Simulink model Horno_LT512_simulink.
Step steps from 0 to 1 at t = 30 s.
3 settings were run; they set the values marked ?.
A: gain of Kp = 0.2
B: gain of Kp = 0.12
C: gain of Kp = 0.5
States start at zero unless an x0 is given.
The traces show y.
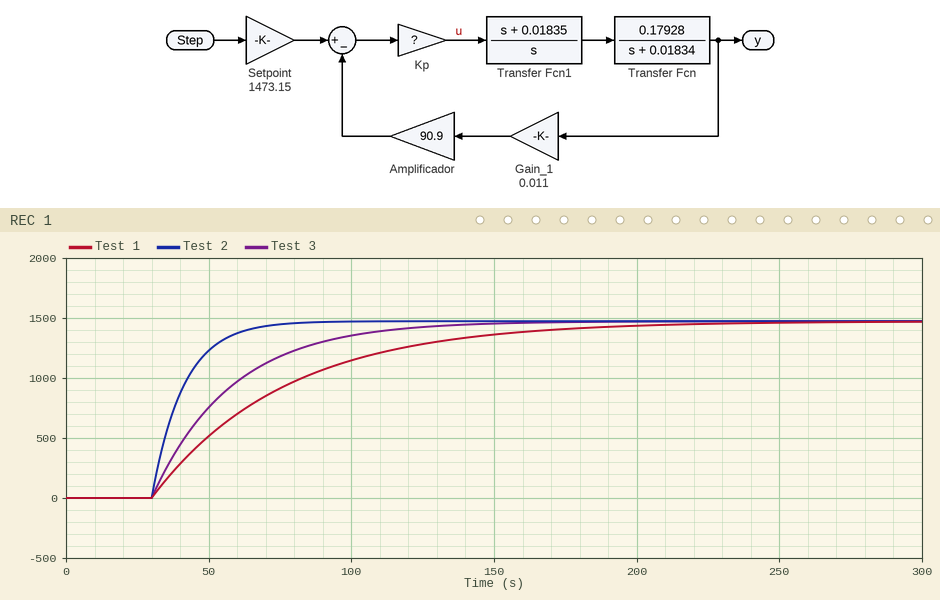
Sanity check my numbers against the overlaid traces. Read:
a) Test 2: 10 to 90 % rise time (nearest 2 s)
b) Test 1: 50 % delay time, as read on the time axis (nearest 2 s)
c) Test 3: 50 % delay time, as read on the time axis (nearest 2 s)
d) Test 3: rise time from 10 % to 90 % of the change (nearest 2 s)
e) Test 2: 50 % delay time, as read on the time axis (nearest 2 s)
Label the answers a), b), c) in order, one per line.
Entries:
a) 24 s
b) 62 s
c) 50 s
d) 62 s
e) 38 s
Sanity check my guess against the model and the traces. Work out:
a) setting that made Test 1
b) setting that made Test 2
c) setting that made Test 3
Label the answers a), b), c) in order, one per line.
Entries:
a) B
b) C
c) A
